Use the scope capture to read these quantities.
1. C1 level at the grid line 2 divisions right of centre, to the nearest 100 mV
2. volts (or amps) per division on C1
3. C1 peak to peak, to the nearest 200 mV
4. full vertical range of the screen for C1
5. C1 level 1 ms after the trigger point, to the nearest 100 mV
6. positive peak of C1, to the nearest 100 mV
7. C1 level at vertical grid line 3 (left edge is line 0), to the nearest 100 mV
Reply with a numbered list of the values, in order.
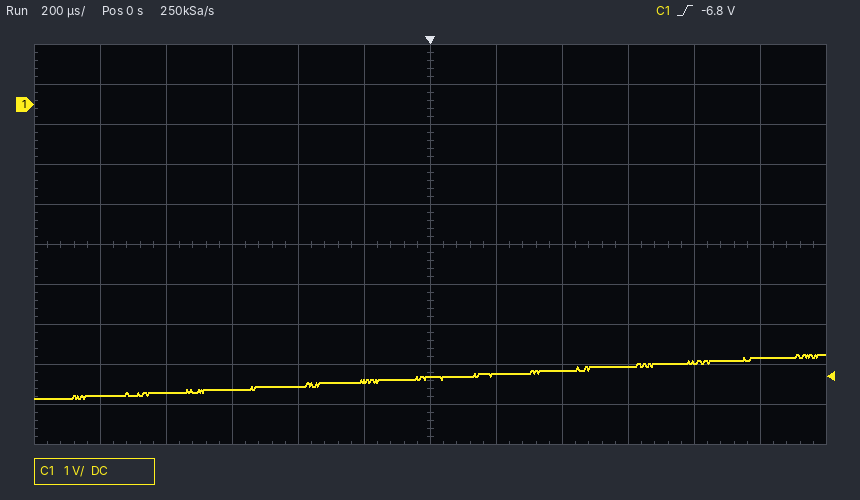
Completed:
1. -6.6 V
2. 1 V
3. 1.2 V
4. 10 V
5. -6.3 V
6. -6.2 V
7. -7.1 V
